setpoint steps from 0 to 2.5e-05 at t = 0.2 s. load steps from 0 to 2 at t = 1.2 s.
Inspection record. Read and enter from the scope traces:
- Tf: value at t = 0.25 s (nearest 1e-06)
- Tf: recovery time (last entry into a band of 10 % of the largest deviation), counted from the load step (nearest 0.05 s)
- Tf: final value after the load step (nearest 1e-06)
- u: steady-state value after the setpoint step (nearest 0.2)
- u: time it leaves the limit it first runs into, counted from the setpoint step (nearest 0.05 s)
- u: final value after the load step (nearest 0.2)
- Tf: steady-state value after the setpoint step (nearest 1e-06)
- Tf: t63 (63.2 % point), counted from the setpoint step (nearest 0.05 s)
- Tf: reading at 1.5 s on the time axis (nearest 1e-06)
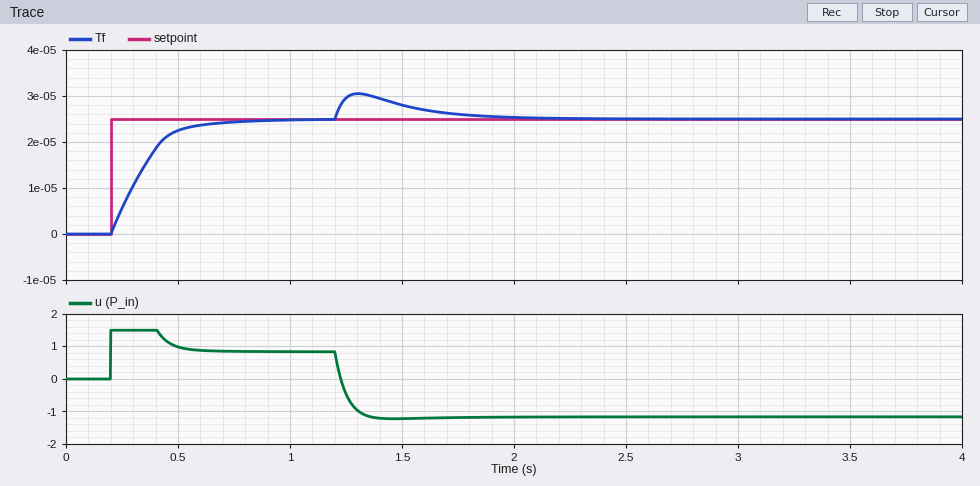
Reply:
0.000006
0.70 s
0.000025
0.8
0.20 s
-1.2
0.000025
0.15 s
0.000028
